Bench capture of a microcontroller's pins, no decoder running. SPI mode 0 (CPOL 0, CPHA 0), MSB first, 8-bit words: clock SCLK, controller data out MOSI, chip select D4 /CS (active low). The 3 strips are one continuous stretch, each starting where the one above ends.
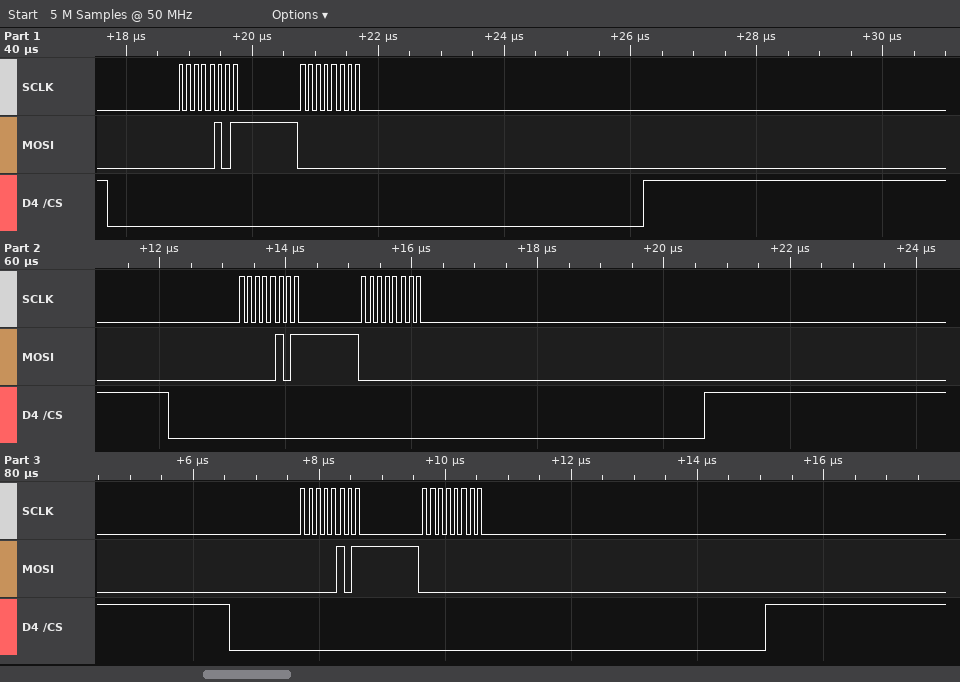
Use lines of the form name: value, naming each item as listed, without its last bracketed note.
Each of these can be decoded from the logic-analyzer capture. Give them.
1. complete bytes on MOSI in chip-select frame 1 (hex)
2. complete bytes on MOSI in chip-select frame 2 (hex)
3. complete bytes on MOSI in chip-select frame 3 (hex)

complete bytes on MOSI in chip-select frame 1: 05 00
complete bytes on MOSI in chip-select frame 2: 05 00
complete bytes on MOSI in chip-select frame 3: 05 00
